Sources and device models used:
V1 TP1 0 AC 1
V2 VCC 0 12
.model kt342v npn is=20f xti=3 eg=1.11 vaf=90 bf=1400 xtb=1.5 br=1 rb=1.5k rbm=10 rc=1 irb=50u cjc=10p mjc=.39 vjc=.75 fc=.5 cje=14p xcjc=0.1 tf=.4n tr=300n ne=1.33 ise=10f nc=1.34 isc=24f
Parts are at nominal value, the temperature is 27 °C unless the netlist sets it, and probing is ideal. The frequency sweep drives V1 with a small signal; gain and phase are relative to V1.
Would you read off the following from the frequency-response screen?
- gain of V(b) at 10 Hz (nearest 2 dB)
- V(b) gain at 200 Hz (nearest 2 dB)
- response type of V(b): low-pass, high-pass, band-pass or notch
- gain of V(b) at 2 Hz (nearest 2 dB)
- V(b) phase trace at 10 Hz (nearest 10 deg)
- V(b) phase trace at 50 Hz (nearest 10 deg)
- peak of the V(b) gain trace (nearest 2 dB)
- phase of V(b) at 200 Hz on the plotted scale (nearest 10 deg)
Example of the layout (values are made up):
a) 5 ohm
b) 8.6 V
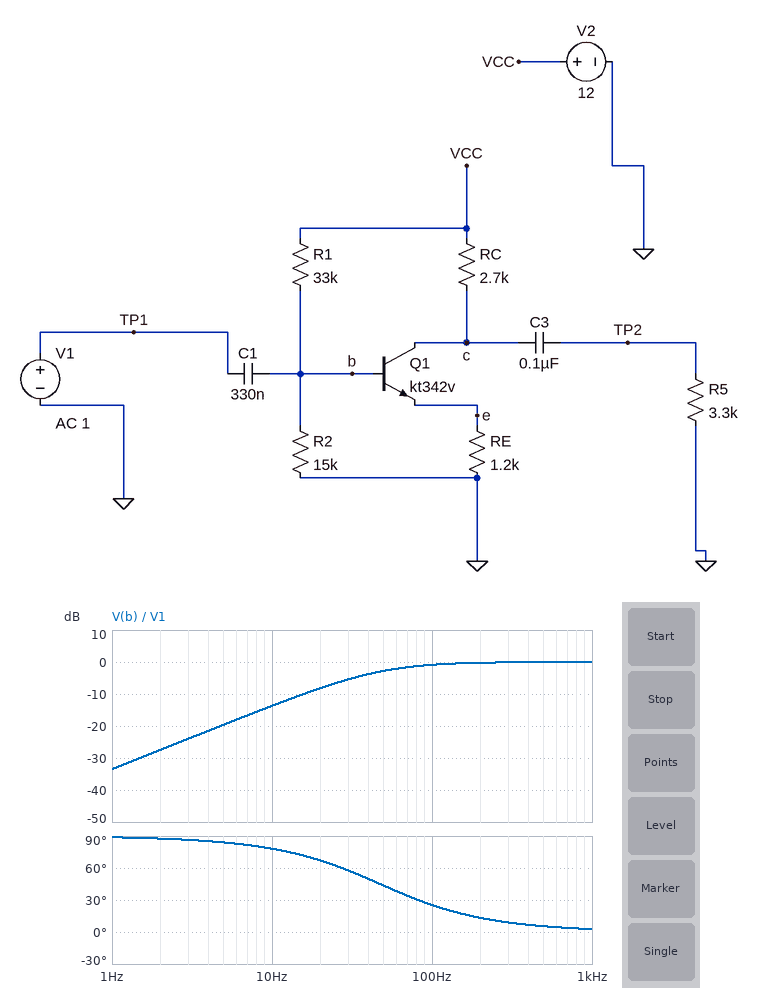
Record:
a) -14 dB
b) 0 dB
c) high-pass
d) -28 dB
e) 80 deg
f) 40 deg
g) 0 dB
h) 10 deg
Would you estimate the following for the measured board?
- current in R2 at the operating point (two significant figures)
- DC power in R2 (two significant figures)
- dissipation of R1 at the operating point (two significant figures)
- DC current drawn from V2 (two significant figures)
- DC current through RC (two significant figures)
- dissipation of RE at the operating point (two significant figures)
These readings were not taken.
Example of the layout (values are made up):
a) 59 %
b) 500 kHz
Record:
a) 250 µA
b) 920 µW
c) 2.1 mW
d) 2.8 mA
e) 2.5 mA
f) 7.7 mW
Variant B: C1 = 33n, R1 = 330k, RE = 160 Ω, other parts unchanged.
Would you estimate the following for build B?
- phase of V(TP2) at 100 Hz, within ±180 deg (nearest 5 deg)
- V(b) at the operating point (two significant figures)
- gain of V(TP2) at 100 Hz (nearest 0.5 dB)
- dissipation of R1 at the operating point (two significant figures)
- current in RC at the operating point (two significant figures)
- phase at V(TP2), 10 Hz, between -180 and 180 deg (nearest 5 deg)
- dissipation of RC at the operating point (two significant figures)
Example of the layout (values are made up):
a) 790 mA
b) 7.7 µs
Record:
a) -35 deg
b) 520 mV
c) -24.0 dB
d) 400 µW
e) 12 µA
f) -5 deg
g) 370 nW
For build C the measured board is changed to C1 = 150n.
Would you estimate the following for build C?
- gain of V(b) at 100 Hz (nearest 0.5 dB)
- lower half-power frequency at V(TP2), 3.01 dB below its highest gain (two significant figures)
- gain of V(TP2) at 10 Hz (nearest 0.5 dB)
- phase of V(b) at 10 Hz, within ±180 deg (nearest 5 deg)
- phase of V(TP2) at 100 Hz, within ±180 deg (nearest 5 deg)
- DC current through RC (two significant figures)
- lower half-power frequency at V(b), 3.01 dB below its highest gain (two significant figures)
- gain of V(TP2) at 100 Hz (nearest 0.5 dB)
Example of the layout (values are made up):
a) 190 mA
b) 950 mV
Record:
a) -3.0 dB
b) 300 Hz
c) -47.0 dB
d) 85 deg
e) -65 deg
f) 2.5 mA
g) 100 Hz
h) -10.5 dB
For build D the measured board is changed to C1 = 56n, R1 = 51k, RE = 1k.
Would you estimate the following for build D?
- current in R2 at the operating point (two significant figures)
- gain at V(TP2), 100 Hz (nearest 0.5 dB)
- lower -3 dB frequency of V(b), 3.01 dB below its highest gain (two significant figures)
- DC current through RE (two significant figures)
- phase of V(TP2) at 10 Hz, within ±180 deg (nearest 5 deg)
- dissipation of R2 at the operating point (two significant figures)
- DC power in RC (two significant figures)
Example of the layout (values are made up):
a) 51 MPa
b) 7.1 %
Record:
a) 180 µA
b) -14.5 dB
c) 250 Hz
d) 2.0 mA
e) -5 deg
f) 480 µW
g) 11 mW
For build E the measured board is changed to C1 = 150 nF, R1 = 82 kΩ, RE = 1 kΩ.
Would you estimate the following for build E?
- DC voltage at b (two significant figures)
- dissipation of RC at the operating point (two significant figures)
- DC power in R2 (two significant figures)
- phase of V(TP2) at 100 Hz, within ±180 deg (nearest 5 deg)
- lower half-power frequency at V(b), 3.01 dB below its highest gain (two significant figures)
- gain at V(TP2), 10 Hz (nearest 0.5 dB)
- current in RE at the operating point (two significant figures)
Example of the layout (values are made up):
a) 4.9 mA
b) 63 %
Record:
a) 1.8 V
b) 3.8 mW
c) 220 µW
d) -70 deg
e) 85 Hz
f) -44.0 dB
g) 1.2 mA
